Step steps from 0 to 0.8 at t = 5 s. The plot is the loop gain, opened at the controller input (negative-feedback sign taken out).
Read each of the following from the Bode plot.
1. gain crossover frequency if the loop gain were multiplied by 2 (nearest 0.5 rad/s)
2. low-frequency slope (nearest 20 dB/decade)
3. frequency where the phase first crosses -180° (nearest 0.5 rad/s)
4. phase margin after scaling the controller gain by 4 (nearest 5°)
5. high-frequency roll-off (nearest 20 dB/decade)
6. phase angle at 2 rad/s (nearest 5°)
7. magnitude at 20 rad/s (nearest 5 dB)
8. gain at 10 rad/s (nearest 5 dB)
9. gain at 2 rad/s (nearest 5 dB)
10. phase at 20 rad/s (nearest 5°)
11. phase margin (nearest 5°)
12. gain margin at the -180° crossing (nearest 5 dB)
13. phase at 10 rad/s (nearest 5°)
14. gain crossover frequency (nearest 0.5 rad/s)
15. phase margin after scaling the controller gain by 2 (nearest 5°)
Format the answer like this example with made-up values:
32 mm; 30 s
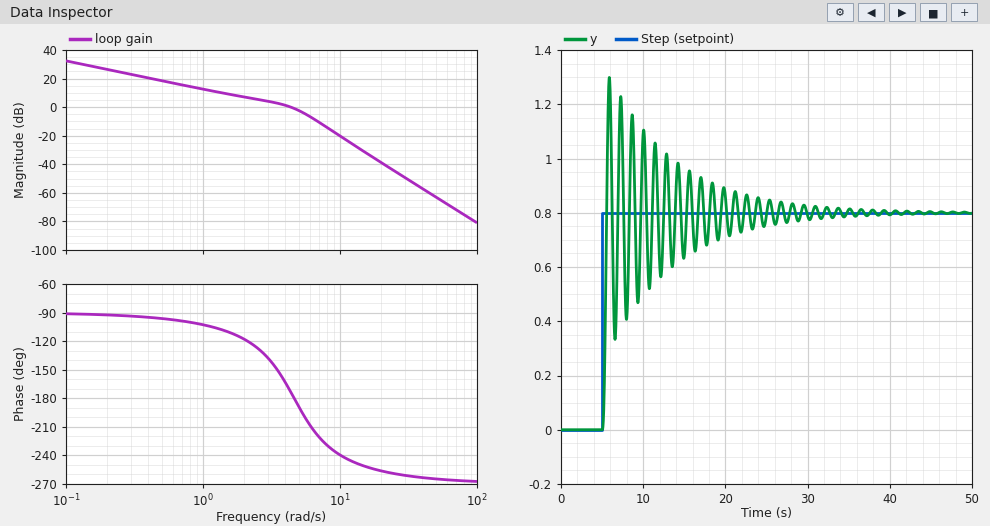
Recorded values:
6.0 rad/s; -20 dB/decade; 4.5 rad/s; -45°; -60 dB/decade; -120°; -40 dB; -20 dB; 5 dB; -255°; 5°; 0 dB; -240°; 4.5 rad/s; -25°
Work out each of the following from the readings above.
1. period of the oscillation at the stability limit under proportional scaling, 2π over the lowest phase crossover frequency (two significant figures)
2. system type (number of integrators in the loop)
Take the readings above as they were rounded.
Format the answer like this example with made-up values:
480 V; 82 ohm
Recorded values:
1.4 s; 1
